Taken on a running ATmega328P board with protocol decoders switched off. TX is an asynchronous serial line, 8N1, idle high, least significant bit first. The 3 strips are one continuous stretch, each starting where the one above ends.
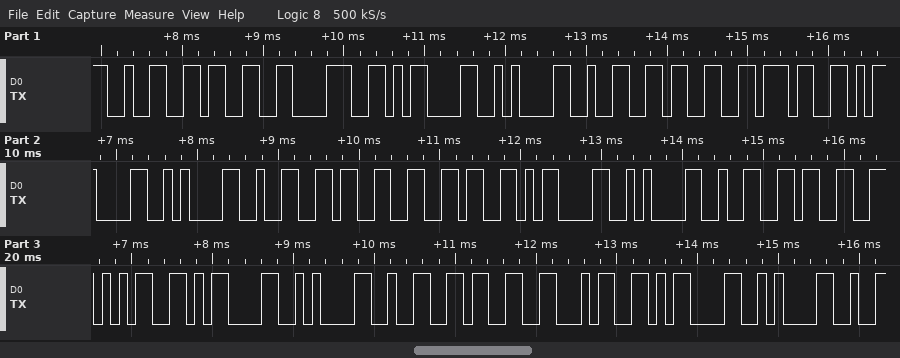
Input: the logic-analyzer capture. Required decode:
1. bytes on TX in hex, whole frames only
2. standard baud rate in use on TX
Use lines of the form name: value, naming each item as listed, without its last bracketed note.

bytes on TX in hex, whole frames only: 32 33 38 0D 0A 32 33 37 0D 0A 32 33 36 0D 0A 32 33 35 0D 0A 32 33 34 0D 0A
standard baud rate in use on TX: 9600 baud
